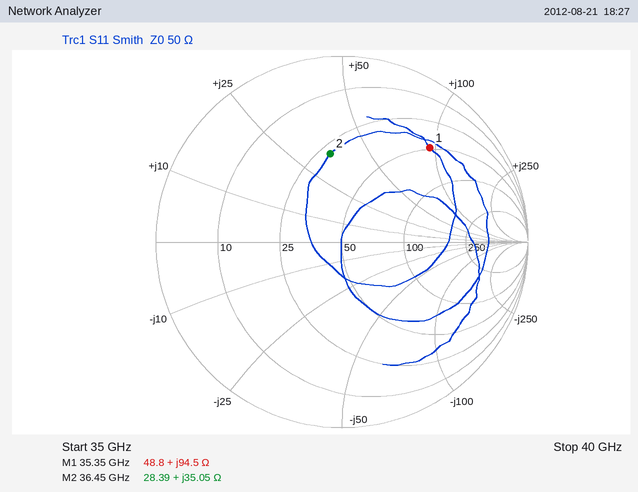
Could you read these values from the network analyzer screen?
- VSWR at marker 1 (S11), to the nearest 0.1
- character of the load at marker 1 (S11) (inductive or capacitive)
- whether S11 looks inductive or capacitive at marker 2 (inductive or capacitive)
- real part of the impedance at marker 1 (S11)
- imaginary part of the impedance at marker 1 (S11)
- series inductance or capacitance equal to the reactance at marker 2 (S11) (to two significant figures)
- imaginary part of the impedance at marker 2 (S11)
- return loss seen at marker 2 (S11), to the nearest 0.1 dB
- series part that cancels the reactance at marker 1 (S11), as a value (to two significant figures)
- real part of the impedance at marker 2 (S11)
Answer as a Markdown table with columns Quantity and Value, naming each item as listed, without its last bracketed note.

| Quantity | Value |
|---|---|
| VSWR at marker 1 (S11), to the nearest 0.1 | 5.5 |
| character of the load at marker 1 (S11) | inductive |
| whether S11 looks inductive or capacitive at marker 2 | inductive |
| real part of the impedance at marker 1 | 48.8 Ω |
| imaginary part of the impedance at marker 1 | +94.5 Ω |
| series inductance or capacitance equal to the reactance at marker 2 (S11) | 150 pH |
| imaginary part of the impedance at marker 2 | +35.05 Ω |
| return loss seen at marker 2 (S11), to the nearest 0.1 dB | 6.4 dB |
| series part that cancels the reactance at marker 1 (S11), as a value | 48 fF |
| real part of the impedance at marker 2 | 28.39 Ω |
